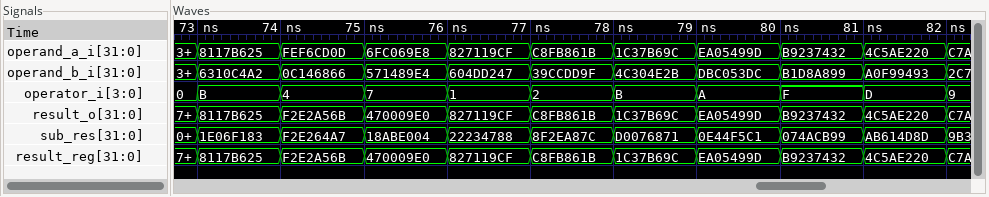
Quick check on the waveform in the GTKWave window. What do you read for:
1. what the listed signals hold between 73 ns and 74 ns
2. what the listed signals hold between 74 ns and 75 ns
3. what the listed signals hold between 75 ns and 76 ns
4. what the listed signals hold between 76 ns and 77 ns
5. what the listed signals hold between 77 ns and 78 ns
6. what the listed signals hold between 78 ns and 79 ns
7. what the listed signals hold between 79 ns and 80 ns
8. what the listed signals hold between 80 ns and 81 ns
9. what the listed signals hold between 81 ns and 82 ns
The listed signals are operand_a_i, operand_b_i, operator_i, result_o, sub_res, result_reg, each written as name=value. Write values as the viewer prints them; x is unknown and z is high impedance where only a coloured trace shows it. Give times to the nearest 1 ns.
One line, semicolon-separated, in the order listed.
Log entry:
operand_a_i=8117B625, operand_b_i=6310C4A2, operator_i=B, result_o=8117B625, sub_res=1E06F183, result_reg=8117B625; operand_a_i=FEF6CD0D, operand_b_i=0C146866, operator_i=4, result_o=F2E2A56B, sub_res=F2E264A7, result_reg=F2E2A56B; operand_a_i=6FC069E8, operand_b_i=571489E4, operator_i=7, result_o=470009E0, sub_res=18ABE004, result_reg=470009E0; operand_a_i=827119CF, operand_b_i=604DD247, operator_i=1, result_o=827119CF, sub_res=22234788, result_reg=827119CF; operand_a_i=C8FB861B, operand_b_i=39CCDD9F, operator_i=2, result_o=C8FB861B, sub_res=8F2EA87C, result_reg=C8FB861B; operand_a_i=1C37B69C, operand_b_i=4C304E2B, operator_i=B, result_o=1C37B69C, sub_res=D0076871, result_reg=1C37B69C; operand_a_i=EA05499D, operand_b_i=DBC053DC, operator_i=A, result_o=EA05499D, sub_res=0E44F5C1, result_reg=EA05499D; operand_a_i=B9237432, operand_b_i=B1D8A899, operator_i=F, result_o=B9237432, sub_res=074ACB99, result_reg=B9237432; operand_a_i=4C5AE220, operand_b_i=A0F99493, operator_i=D, result_o=4C5AE220, sub_res=AB614D8D, result_reg=4C5AE220
